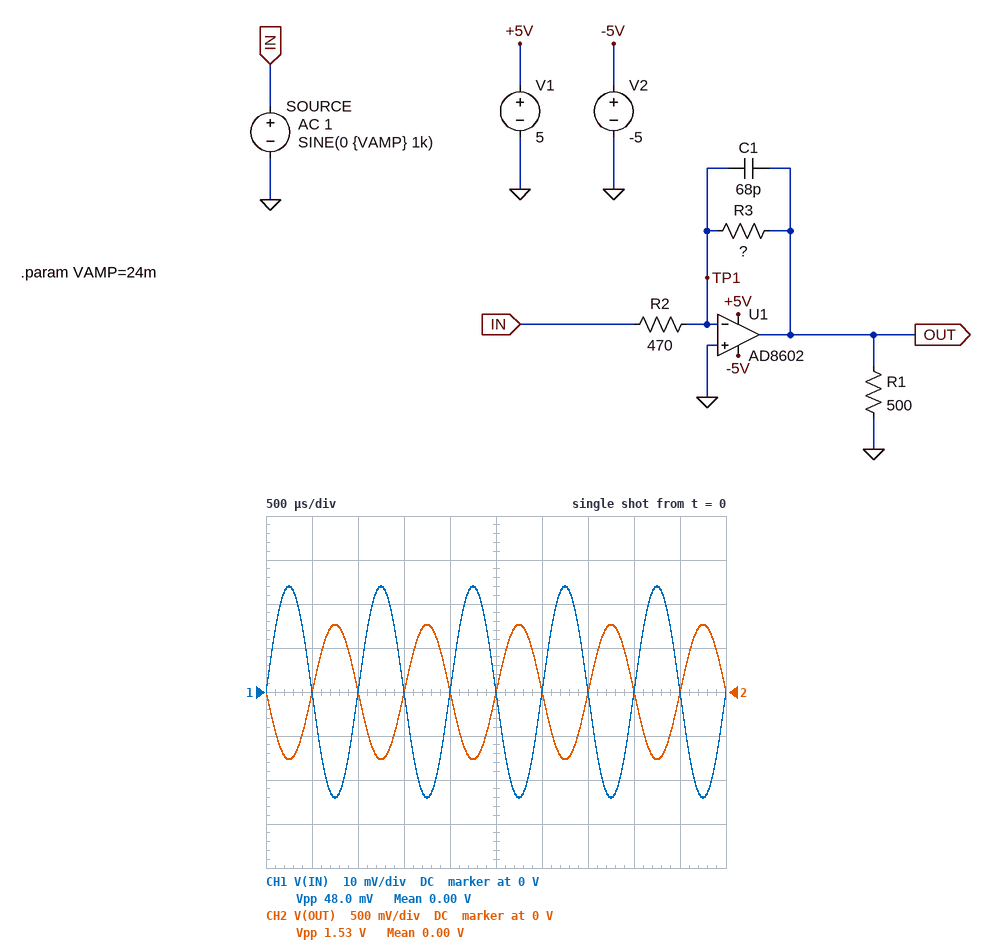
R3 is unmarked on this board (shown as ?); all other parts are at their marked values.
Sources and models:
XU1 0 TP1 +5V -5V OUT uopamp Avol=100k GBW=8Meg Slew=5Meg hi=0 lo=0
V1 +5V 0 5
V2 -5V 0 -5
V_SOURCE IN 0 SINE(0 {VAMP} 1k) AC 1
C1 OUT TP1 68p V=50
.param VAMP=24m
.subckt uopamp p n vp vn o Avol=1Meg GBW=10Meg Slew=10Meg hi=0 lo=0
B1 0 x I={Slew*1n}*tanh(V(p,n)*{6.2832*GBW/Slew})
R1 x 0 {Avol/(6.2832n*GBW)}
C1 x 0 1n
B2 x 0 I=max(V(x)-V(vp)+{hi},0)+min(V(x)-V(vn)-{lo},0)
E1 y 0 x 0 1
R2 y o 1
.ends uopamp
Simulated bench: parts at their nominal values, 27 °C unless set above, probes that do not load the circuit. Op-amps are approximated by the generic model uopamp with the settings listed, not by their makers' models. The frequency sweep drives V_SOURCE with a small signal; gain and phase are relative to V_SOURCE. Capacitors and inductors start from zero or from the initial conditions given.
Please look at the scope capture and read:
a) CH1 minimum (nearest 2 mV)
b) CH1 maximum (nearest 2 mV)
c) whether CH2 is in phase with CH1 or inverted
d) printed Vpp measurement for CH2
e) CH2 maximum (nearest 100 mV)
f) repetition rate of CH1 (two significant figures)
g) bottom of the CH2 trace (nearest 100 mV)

-24 mV
24 mV
inverted
1.53 V
800 mV
1.0 kHz
-800 mV
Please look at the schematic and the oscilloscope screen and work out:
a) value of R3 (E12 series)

15 kΩ
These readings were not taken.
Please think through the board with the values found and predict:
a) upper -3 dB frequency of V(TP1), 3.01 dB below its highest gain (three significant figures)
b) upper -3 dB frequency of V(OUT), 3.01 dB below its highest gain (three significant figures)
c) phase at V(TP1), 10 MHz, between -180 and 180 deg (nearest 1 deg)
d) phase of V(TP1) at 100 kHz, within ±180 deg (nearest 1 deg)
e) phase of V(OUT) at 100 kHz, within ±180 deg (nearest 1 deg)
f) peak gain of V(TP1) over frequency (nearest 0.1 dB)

13.2 MHz
95.7 kHz
-37 deg
43 deg
133 deg
-8.4 dB
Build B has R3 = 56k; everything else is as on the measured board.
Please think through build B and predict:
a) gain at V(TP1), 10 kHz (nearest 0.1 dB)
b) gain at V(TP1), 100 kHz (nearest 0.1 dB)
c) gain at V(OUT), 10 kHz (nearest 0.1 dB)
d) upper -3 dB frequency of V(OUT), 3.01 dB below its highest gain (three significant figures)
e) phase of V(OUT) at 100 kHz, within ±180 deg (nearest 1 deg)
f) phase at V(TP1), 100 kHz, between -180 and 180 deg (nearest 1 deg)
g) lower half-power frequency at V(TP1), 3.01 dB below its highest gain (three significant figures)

-17.1 dB
-8.6 dB
40.9 dB
25.7 kHz
104 deg
14 deg
25.6 kHz
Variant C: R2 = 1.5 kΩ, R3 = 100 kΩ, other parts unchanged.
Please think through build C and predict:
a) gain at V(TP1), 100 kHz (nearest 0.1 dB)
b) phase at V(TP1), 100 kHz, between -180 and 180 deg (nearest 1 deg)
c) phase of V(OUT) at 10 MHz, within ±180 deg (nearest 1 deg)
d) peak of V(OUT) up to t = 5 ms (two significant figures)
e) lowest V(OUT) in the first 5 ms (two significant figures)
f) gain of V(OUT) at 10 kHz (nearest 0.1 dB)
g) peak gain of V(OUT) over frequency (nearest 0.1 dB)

-15.9 dB
10 deg
44 deg
1.6 V
-1.6 V
35.5 dB
36.5 dB
